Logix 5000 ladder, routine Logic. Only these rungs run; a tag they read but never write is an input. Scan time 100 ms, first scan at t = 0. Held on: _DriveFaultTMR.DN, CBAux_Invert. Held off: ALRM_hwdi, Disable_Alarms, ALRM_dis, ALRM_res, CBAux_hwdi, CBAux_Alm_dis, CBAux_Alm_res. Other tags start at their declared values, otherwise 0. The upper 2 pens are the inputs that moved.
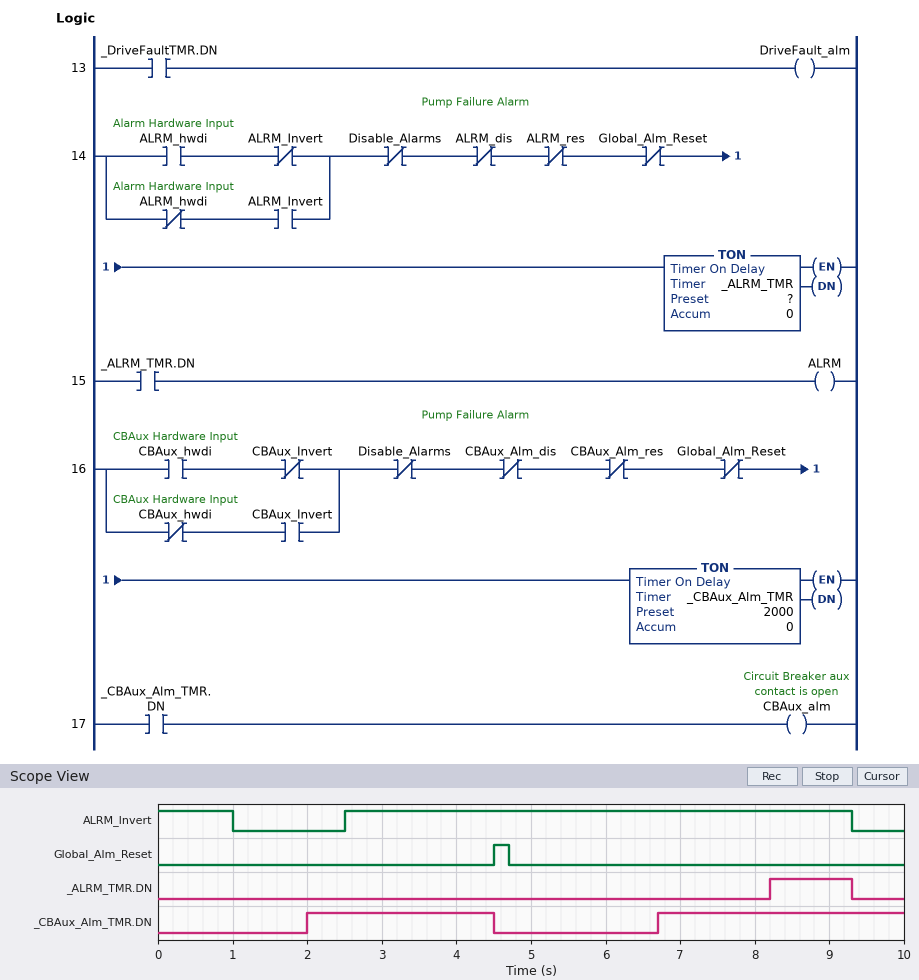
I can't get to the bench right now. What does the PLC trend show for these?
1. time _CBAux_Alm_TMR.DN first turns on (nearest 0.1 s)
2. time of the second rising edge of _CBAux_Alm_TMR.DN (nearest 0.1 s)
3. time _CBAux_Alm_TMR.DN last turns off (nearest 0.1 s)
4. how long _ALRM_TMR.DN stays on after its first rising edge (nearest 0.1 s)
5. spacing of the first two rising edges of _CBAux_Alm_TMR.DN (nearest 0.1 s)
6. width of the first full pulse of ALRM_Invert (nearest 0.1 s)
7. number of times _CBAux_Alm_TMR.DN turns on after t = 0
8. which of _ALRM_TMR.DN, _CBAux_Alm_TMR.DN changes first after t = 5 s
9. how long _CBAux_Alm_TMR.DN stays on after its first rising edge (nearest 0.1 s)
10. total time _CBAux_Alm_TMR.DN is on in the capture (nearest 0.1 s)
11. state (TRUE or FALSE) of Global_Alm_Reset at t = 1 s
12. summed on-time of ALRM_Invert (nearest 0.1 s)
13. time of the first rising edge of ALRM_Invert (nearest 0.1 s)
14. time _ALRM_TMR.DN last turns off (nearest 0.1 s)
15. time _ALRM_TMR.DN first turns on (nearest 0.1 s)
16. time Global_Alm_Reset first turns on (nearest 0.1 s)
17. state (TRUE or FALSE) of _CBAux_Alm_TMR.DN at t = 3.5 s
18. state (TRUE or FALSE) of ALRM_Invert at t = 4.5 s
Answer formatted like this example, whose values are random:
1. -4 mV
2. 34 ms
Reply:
1. 2.0 s
2. 6.7 s
3. 4.5 s
4. 1.1 s
5. 4.7 s
6. 6.8 s
7. 2
8. _CBAux_Alm_TMR.DN
9. 2.5 s
10. 5.8 s
11. FALSE
12. 7.8 s
13. 2.5 s
14. 9.3 s
15. 8.2 s
16. 4.5 s
17. TRUE
18. TRUE
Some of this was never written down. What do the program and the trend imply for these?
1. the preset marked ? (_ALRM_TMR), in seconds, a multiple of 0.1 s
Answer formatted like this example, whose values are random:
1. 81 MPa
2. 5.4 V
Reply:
1. 3.5 s
